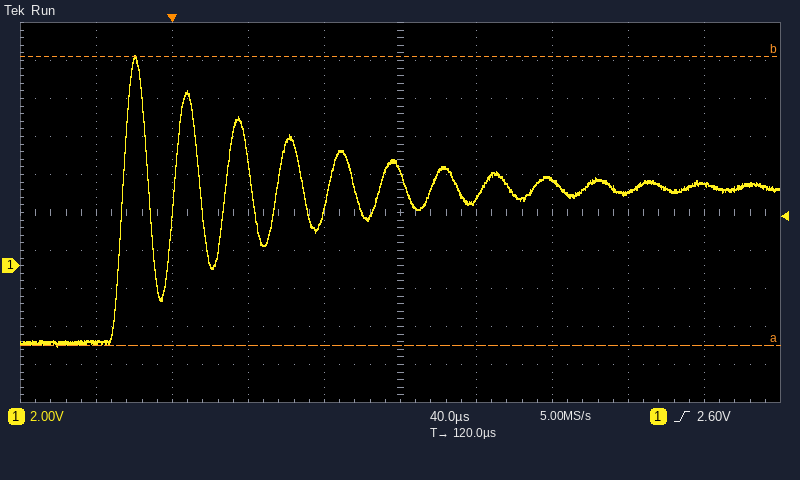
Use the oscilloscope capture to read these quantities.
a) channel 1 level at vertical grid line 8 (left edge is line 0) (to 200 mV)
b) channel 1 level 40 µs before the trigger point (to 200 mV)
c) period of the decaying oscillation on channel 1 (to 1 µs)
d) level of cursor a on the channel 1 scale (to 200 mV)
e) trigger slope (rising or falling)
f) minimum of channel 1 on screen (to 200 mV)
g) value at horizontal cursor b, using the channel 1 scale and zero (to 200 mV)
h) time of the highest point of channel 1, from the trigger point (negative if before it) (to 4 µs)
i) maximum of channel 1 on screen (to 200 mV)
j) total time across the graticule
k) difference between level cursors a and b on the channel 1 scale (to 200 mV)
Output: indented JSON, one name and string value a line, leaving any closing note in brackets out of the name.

{
  "channel 1 level at vertical grid line 8 (left edge is line 0)": "3.8 V",
  "channel 1 level 40 µs before the trigger point": "-4.0 V",
  "period of the decaying oscillation on channel 1": "27 µs",
  "level of cursor a on the channel 1 scale": "-4.2 V",
  "trigger slope": "rising",
  "minimum of channel 1 on screen": "-4.2 V",
  "value at horizontal cursor b, using the channel 1 scale and zero": "11.0 V",
  "time of the highest point of channel 1, from the trigger point (negative if before it)": "-20 µs",
  "maximum of channel 1 on screen": "11.0 V",
  "total time across the graticule": "400 µs",
  "difference between level cursors a and b on the channel 1 scale": "15.2 V"
}
